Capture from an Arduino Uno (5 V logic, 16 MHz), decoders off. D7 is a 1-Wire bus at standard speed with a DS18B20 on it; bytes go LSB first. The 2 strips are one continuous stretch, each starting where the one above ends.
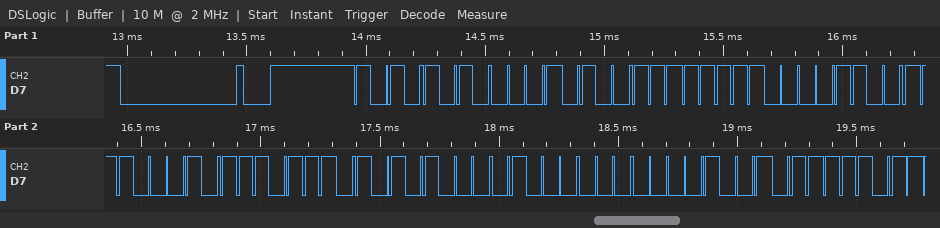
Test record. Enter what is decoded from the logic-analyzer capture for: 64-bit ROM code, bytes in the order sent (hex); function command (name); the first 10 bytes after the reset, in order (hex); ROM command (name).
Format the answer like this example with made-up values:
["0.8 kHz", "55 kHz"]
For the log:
["28 FF 30 47 77 15 02 90", "Read Scratchpad", "55 28 FF 30 47 77 15 02 90 BE", "Match ROM"]
